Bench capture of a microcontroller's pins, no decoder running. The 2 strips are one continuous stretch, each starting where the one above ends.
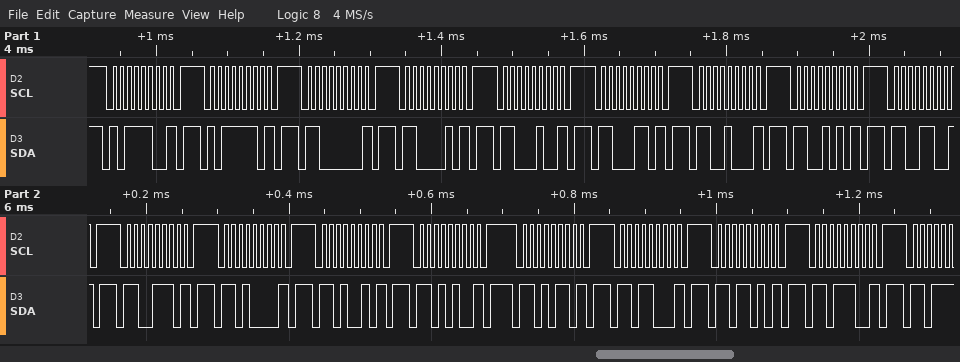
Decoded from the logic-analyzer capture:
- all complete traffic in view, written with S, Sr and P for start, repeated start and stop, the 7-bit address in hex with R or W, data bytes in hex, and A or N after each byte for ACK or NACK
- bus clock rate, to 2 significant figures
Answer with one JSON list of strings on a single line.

["S 5EW N P S 5FW N P S 60W N P S 61W N P S 62W N P S 63W N P S 64W N P S 65W N P S 66W N P S 67W N P S 68W N P S 69W N P S 6AW N P S 6BW N P S 6CW N P S 6DW N P S 6EW N P", "100 kHz"]
